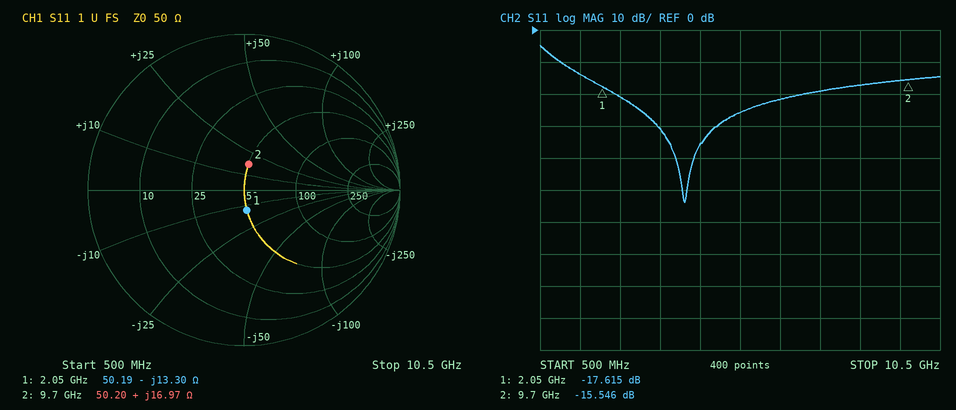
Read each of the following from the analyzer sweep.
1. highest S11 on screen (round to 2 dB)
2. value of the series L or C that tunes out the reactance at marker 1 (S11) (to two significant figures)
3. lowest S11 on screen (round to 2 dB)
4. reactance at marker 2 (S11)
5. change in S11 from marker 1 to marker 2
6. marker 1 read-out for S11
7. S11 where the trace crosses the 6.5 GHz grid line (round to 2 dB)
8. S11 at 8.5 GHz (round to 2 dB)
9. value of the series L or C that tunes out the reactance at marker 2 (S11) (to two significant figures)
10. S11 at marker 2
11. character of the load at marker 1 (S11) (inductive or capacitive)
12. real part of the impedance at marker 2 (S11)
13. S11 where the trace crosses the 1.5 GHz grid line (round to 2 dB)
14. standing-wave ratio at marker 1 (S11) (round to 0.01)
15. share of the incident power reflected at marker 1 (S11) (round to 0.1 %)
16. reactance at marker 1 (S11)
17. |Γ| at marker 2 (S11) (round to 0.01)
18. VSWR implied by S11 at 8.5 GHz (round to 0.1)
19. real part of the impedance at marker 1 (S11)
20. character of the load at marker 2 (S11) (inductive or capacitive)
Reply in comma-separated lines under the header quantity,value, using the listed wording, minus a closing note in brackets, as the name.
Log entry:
quantity,value
highest S11 on screen,-4 dB
value of the series L or C that tunes out the reactance at marker 1 (S11),1.0 nH
lowest S11 on screen,-54 dB
reactance at marker 2,+16.97 Ω
change in S11 from marker 1 to marker 2,2.069 dB
marker 1 read-out for S11,-17.615 dB
S11 where the trace crosses the 6.5 GHz grid line,-22 dB
S11 at 8.5 GHz,-18 dB
value of the series L or C that tunes out the reactance at marker 2 (S11),970 fF
S11 at marker 2,-15.546 dB
character of the load at marker 1 (S11),capacitive
real part of the impedance at marker 2,50.20 Ω
S11 where the trace crosses the 1.5 GHz grid line,-14 dB
standing-wave ratio at marker 1 (S11),1.30
share of the incident power reflected at marker 1 (S11),1.7 %
reactance at marker 1,-13.30 Ω
|Γ| at marker 2 (S11),0.17
VSWR implied by S11 at 8.5 GHz,1.3
real part of the impedance at marker 1,50.19 Ω
character of the load at marker 2 (S11),inductive
